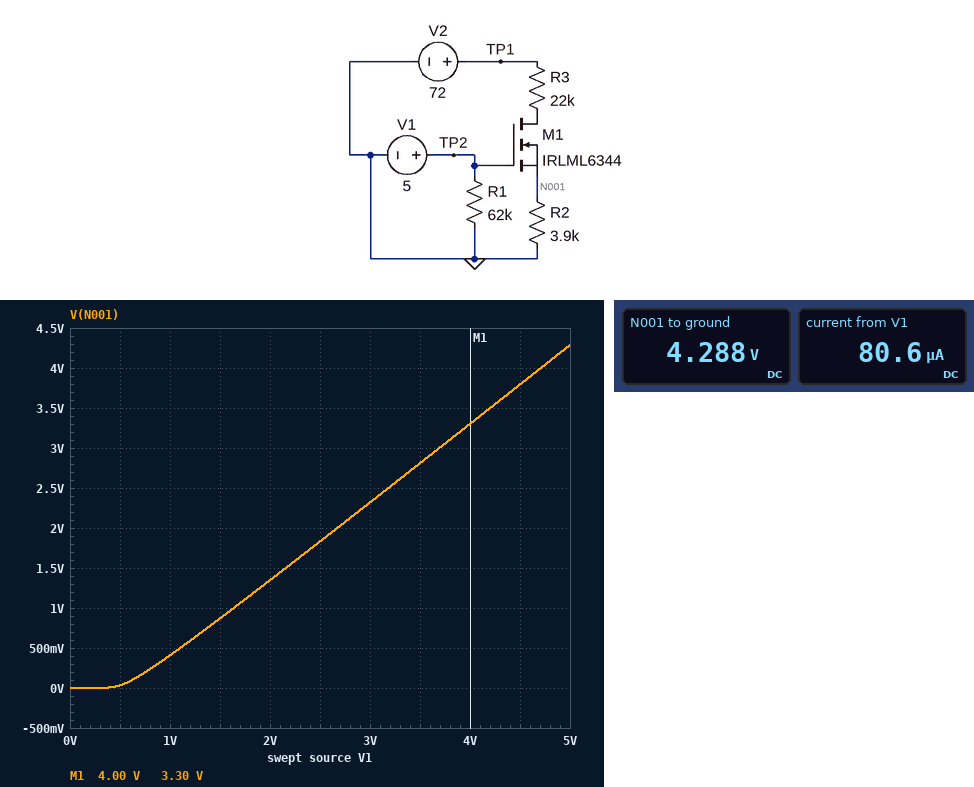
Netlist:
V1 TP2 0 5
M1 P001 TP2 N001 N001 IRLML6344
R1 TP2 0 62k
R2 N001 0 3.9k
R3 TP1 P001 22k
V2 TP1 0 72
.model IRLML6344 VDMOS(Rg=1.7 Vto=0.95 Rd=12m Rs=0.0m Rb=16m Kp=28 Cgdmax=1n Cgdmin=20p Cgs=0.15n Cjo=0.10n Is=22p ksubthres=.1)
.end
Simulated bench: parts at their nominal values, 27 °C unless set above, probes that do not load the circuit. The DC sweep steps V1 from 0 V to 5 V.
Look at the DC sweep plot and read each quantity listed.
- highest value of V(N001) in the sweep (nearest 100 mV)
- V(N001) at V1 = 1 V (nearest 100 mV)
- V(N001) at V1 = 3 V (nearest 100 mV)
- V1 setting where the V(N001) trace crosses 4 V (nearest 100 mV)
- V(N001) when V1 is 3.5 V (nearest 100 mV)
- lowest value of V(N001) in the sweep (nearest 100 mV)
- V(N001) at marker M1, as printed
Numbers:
4.3 V
400 mV
2.3 V
4.7 V
2.8 V
0 V
3.30 V
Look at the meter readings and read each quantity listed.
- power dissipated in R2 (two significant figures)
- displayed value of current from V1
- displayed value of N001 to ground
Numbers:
4.7 mW
80.6 µA
4.288 V
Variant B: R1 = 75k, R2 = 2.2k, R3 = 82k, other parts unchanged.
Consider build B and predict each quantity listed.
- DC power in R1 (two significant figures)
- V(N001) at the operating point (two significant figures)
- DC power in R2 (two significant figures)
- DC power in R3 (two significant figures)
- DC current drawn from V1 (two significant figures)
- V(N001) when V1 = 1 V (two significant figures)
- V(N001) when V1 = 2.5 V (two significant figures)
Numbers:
330 µW
1.9 V
1.6 mW
60 mW
67 µA
380 mV
1.8 V
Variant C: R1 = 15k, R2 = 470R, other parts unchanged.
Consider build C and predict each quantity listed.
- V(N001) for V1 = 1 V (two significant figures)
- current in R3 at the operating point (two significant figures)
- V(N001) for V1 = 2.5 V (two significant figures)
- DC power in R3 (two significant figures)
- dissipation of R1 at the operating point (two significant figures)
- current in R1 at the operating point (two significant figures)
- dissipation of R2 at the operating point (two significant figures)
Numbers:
310 mV
3.2 mA
1.5 V
230 mW
1.7 mW
330 µA
4.8 mW
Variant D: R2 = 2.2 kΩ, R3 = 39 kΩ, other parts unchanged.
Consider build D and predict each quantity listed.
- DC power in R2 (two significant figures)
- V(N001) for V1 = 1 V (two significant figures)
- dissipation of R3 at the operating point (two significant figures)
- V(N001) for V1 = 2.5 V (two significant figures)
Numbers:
6.7 mW
380 mV
120 mW
1.8 V
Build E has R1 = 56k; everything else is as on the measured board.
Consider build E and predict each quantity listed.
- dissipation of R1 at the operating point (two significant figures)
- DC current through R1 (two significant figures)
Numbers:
450 µW
89 µA
